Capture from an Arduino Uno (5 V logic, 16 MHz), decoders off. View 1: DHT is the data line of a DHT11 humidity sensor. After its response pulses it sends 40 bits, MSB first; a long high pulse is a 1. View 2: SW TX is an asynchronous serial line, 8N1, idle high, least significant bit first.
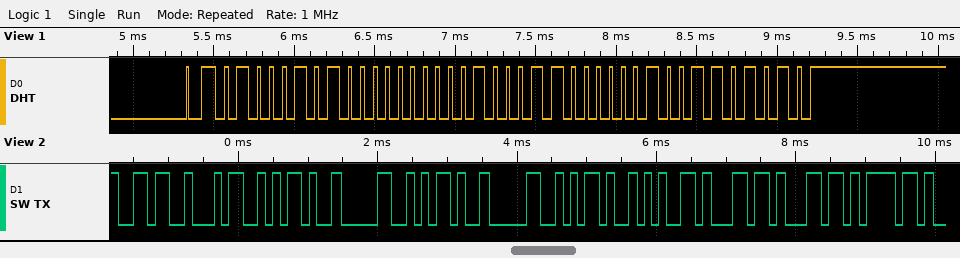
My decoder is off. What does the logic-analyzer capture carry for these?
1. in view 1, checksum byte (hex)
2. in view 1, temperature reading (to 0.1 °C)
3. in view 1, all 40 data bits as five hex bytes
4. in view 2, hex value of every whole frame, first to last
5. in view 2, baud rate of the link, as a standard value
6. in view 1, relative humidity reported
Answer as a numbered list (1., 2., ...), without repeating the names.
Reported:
1. 0x6A
2. 35.2 °C
3. 45 00 23 02 6A
4. 36 34 2D 30 2D 30 2D 65 6C 6C 6F
5. 9600 baud
6. 69 %
